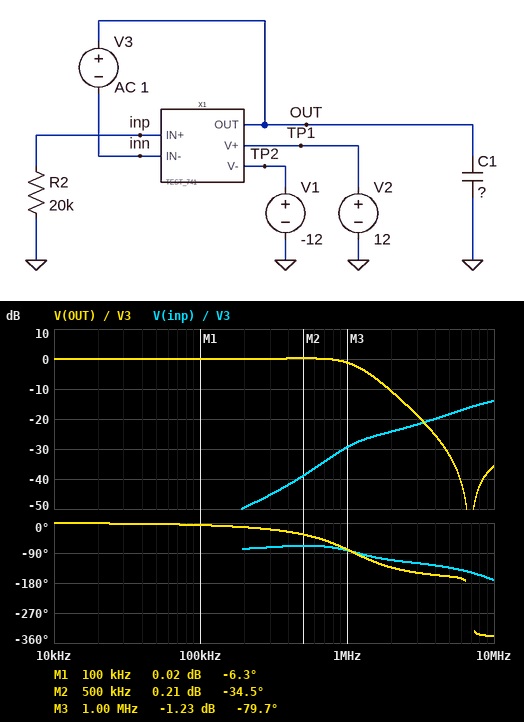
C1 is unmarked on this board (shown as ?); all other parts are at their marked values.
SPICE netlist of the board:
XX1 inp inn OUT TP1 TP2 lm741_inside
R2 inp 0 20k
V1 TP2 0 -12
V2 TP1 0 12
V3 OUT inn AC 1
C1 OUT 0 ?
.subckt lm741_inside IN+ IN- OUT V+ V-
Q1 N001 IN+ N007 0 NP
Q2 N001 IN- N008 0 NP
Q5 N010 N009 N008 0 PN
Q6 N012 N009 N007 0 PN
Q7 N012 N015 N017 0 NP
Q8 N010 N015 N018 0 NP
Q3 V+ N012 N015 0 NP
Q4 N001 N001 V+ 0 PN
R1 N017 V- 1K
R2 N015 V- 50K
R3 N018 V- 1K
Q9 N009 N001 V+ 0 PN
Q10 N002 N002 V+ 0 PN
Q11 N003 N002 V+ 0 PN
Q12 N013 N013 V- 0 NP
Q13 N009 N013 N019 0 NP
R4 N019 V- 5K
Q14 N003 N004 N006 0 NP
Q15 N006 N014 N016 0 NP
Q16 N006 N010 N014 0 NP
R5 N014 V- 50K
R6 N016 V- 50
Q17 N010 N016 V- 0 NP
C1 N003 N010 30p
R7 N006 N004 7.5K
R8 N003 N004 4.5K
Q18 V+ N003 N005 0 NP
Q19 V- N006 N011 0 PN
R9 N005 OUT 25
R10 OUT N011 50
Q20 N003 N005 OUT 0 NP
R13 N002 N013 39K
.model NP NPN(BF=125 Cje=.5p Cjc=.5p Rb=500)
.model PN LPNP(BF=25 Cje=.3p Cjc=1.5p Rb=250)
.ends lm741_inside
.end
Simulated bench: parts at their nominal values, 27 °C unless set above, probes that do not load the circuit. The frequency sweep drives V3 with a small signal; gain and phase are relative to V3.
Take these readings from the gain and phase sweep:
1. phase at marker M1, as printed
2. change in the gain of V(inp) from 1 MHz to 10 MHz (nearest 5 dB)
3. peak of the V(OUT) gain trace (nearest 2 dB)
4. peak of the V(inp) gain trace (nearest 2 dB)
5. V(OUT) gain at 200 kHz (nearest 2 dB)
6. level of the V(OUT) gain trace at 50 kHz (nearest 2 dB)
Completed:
-6.3 deg
15 dB
0 dB
-14 dB
0 dB
0 dB
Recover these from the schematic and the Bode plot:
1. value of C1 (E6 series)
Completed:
15 pF
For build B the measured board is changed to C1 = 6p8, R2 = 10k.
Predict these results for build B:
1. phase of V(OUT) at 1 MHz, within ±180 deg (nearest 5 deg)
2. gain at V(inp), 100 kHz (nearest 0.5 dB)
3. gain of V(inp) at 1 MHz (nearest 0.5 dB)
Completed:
-60 deg
-62.0 dB
-37.5 dB
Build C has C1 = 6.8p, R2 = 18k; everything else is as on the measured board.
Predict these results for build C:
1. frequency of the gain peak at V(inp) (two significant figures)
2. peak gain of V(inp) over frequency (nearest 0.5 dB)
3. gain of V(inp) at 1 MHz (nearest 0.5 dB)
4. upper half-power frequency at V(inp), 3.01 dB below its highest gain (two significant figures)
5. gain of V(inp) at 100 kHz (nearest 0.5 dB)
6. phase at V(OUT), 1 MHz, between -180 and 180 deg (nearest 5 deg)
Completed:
14 MHz
-14.0 dB
-32.5 dB
26 MHz
-57.0 dB
-60 deg
